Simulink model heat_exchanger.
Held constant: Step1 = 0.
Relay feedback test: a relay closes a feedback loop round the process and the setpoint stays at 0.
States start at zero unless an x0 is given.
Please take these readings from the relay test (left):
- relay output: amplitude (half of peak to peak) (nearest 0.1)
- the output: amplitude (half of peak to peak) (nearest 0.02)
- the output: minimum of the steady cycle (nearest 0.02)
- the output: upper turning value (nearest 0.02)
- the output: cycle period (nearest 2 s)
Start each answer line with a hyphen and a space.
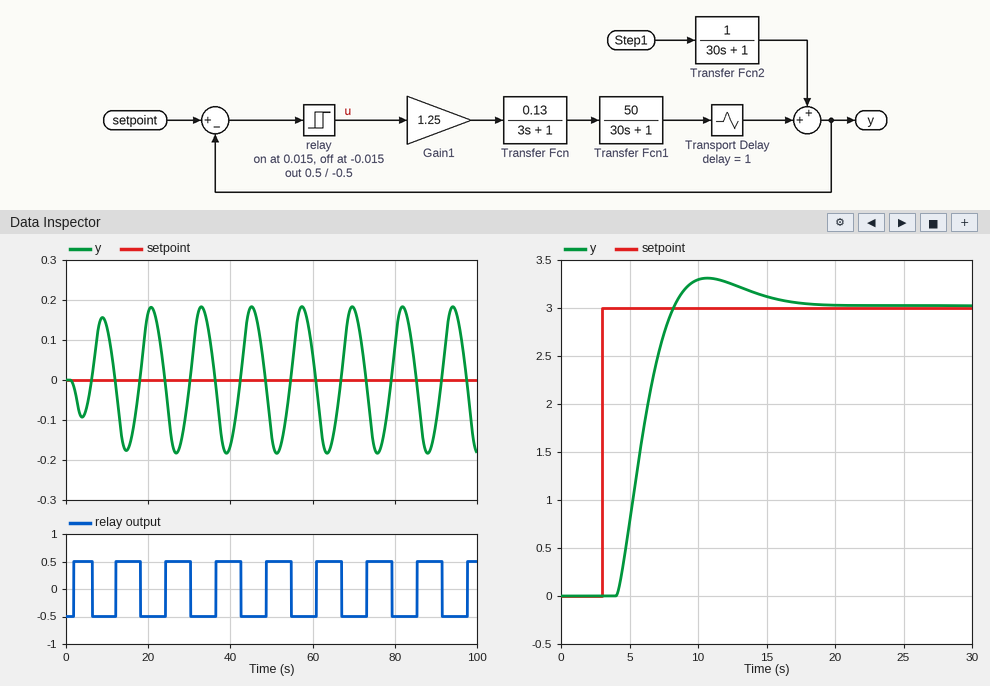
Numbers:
- 0.5
- 0.18
- -0.18
- 0.18
- 12 s
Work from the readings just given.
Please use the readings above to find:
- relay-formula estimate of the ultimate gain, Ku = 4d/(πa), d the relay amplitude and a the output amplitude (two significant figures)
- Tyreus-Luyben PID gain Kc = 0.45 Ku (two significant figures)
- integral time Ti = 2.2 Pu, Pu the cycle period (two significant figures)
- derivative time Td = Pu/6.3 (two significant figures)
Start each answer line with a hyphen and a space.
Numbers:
- 3.5
- 1.6
- 26 s
- 1.9 s
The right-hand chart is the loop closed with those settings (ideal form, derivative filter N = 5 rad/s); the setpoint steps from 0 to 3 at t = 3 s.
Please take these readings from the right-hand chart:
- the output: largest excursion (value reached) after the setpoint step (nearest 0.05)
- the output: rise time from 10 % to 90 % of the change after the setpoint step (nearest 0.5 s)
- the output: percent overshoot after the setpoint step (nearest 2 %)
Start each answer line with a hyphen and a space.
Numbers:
- 3.30
- 3.0 s
- 10 %
